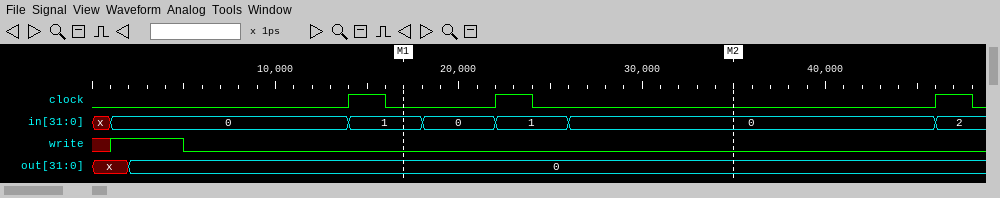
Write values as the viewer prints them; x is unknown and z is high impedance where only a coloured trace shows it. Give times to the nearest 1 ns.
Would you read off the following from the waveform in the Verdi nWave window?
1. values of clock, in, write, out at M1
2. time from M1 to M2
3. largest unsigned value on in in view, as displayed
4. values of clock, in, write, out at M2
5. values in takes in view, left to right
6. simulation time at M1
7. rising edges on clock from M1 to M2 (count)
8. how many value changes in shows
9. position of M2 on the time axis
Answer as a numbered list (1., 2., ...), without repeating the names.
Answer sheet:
1. clock=0, in=1, write=0, out=0
2. 18 ns
3. 2
4. clock=0, in=0, write=0, out=0
5. x, 0, 1, 0, 1, 0, 2
6. 17 ns
7. 1
8. 6
9. 35 ns
